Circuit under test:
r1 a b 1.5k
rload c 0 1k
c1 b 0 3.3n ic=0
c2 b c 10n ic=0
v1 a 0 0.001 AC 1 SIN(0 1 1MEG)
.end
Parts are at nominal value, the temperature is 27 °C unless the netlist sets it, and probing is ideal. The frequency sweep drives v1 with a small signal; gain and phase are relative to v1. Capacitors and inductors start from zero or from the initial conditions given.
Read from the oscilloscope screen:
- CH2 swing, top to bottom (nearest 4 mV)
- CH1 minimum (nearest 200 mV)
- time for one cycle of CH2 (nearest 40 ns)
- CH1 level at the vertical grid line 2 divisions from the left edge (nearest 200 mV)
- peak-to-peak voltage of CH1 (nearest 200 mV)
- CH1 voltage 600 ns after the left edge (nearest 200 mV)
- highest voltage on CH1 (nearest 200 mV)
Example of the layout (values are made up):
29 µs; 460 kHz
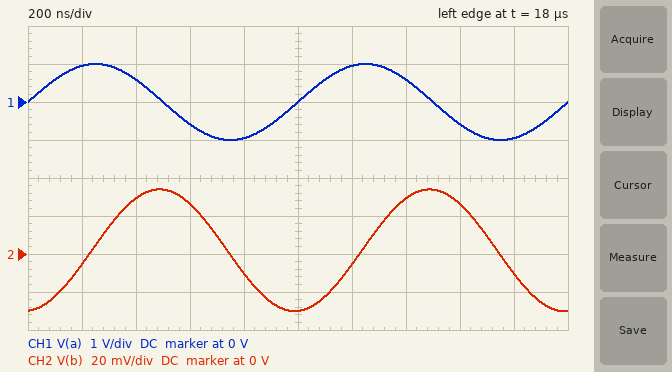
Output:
64 mV; -1.0 V; 1.00 µs; 600 mV; 2.0 V; -600 mV; 1.0 V
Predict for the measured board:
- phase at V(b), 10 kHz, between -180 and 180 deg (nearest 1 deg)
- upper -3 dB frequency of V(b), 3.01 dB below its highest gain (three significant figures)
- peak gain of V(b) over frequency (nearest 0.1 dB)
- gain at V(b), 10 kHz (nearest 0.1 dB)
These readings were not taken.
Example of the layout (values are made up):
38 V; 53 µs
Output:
-35 deg; 6.49 kHz; 0 dB; -4.8 dB
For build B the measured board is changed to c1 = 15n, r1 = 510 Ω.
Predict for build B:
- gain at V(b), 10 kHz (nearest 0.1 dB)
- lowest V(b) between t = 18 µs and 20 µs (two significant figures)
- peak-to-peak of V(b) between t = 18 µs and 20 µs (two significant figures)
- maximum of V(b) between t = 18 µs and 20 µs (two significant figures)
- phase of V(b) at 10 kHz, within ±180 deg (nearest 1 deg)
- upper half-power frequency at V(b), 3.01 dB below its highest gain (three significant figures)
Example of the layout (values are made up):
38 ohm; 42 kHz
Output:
-2.6 dB; -19 mV; 42 mV; 23 mV; -32 deg; 11.4 kHz
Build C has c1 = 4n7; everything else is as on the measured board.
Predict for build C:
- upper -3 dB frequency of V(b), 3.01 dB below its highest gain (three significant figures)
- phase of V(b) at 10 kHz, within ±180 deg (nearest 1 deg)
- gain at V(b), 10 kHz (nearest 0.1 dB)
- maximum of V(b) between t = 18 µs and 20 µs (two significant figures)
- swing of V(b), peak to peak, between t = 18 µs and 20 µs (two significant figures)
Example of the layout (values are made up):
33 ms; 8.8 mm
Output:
6.04 kHz; -38 deg; -5.2 dB; 25 mV; 45 mV
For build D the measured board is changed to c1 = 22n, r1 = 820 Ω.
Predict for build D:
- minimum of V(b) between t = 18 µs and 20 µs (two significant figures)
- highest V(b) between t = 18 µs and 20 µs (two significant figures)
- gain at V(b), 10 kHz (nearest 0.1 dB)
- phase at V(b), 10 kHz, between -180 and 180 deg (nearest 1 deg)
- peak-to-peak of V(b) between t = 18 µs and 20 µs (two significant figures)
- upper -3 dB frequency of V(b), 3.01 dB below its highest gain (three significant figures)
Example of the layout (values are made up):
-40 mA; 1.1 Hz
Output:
-6.4 mV; 11 mV; -5.8 dB; -51 deg; 18 mV; 5.65 kHz
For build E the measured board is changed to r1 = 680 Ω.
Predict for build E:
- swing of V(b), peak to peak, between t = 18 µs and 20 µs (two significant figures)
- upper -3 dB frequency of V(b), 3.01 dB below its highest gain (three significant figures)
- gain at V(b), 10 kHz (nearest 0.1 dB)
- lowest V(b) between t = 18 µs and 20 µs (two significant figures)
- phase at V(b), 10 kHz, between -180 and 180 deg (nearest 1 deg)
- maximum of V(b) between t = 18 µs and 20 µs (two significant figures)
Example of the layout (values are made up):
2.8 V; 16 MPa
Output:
140 mV; 14.4 kHz; -2.1 dB; -69 mV; -21 deg; 72 mV
